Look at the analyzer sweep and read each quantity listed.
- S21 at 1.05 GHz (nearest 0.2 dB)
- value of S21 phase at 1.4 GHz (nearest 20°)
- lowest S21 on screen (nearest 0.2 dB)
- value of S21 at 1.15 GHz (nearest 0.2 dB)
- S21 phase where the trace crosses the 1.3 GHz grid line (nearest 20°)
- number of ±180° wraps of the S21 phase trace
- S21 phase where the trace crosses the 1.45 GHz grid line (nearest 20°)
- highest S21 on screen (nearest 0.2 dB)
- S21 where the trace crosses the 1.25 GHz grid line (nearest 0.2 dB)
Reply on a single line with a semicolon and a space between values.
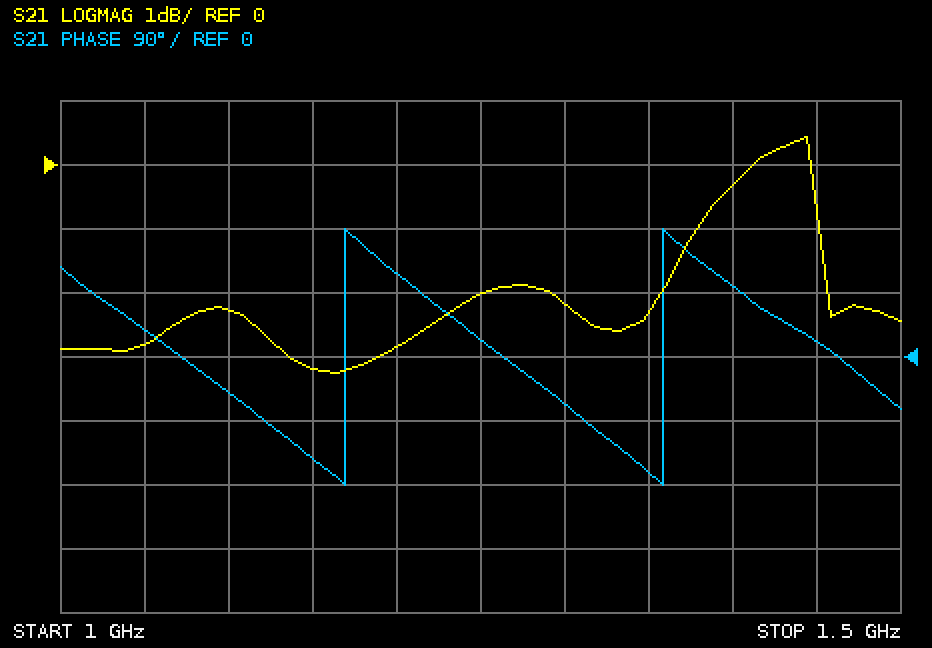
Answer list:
-2.8 dB; 100°; -3.2 dB; -3.2 dB; -60°; 2; 20°; 0.4 dB; -2.0 dB
